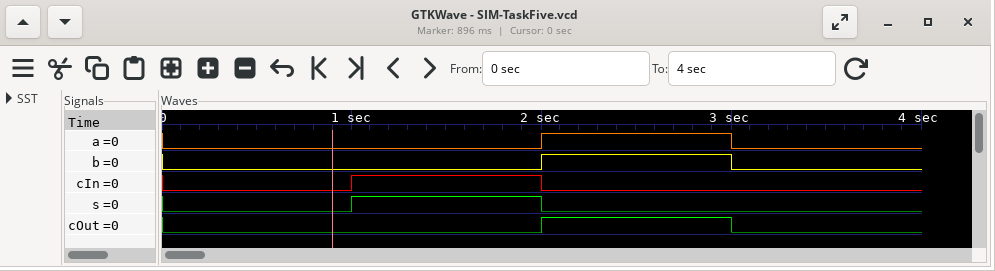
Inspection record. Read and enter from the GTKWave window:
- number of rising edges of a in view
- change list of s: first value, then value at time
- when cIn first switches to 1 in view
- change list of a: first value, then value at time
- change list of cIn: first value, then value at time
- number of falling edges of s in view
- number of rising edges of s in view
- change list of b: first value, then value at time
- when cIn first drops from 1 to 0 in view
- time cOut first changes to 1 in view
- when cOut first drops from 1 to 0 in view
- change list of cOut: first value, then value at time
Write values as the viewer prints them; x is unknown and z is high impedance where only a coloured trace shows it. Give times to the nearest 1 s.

1
0, 1 at 1 s, 0 at 2 s
1 s
0, 1 at 2 s, 0 at 3 s
0, 1 at 1 s, 0 at 2 s
1
1
0, 1 at 2 s, 0 at 3 s
2 s
2 s
3 s
0, 1 at 2 s, 0 at 3 s
